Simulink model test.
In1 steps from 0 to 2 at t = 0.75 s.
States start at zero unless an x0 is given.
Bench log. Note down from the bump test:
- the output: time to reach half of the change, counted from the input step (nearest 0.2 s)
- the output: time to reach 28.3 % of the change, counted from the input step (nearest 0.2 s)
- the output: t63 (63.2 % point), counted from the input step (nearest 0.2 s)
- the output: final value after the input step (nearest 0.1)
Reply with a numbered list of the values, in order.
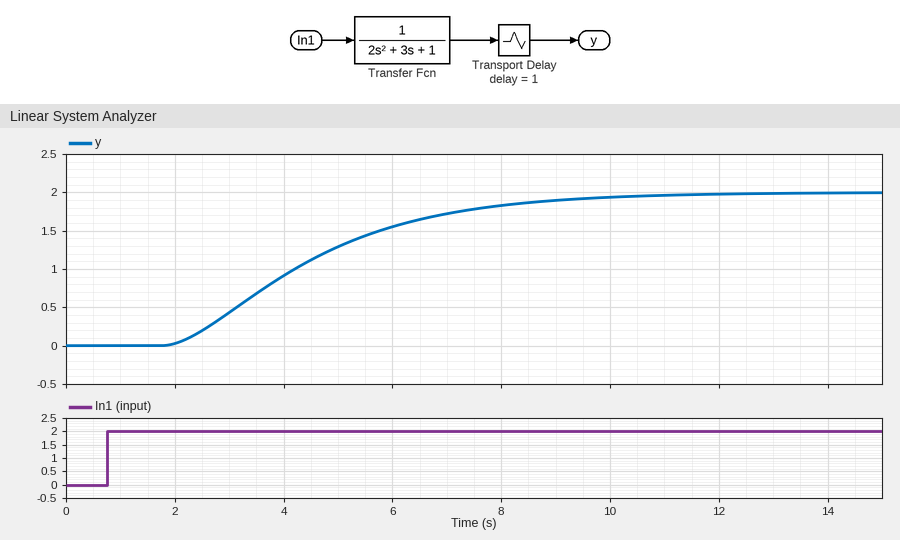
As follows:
1. 3.4 s
2. 2.6 s
3. 4.2 s
4. 2.0
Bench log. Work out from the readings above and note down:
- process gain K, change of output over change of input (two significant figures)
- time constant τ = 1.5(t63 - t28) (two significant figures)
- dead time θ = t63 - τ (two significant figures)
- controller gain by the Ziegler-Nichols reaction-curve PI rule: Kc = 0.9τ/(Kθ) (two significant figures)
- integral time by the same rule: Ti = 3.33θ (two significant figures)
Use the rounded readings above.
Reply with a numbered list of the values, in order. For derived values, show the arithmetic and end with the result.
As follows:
1. (2 - 0) / 2 = 1.0
2. 1.5 × (4.2 - 2.6) = 2.4 s
3. 4.2 - 2.4 = 1.8 s
4. 0.9 × 2.4 / (1 × 1.8) = 1.2
5. 3.33 × 1.8 = 6.0 s
